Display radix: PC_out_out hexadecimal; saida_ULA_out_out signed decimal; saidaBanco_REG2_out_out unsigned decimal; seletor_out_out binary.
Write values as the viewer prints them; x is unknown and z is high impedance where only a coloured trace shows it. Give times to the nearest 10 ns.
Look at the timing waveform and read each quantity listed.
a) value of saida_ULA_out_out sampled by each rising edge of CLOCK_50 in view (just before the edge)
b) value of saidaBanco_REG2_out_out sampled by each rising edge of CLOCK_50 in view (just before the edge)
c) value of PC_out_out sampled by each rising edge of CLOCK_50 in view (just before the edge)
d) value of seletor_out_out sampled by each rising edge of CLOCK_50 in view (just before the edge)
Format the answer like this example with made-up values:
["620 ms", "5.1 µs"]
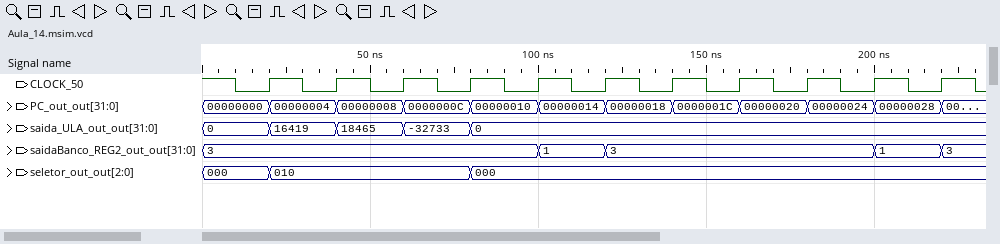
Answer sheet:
["0, 16419, 18465, -32733, 0, 0, 0, 0, 0, 0, 0", "3, 3, 3, 3, 3, 1, 3, 3, 3, 3, 1", "00000000, 00000004, 00000008, 0000000C, 00000010, 00000014, 00000018, 0000001C, 00000020, 00000024, 00000028", "000, 010, 010, 010, 000, 000, 000, 000, 000, 000, 000"]
